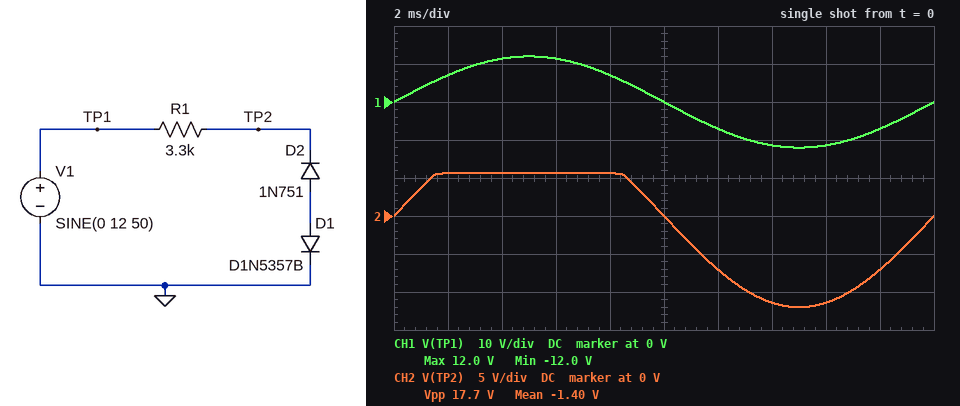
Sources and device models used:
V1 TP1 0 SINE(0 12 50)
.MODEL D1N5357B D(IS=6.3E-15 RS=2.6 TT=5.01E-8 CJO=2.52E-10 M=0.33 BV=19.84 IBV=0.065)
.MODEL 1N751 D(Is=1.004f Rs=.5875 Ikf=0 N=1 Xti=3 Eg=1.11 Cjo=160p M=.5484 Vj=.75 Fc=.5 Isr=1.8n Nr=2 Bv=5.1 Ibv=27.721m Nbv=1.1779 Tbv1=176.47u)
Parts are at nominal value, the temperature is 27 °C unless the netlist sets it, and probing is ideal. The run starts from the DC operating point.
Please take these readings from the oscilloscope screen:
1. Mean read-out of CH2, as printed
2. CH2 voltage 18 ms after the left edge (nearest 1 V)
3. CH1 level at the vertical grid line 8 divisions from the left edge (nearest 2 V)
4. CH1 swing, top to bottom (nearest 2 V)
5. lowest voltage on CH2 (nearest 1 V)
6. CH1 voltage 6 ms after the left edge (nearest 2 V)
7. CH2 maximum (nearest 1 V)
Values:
-1.40 V
-7 V
-12 V
24 V
-12 V
12 V
6 V
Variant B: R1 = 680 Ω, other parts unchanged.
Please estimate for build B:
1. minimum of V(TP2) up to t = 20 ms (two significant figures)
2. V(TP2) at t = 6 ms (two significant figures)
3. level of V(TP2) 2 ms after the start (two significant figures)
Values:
-12 V
5.8 V
5.7 V
